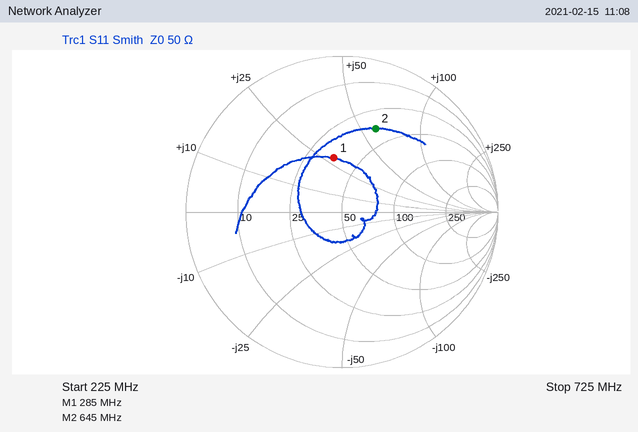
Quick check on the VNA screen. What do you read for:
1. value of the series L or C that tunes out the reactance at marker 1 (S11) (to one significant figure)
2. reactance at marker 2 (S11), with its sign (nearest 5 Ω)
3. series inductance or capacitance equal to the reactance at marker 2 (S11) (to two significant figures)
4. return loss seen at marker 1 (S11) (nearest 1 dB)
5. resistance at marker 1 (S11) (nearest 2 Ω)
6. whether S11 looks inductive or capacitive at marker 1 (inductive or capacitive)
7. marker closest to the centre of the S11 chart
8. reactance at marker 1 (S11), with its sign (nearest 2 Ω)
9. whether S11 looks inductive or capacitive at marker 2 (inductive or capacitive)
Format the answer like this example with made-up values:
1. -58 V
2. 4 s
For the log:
1. 20 pF
2. +60 Ω
3. 15 nH
4. 9 dB
5. 36 Ω
6. inductive
7. marker 1
8. +28 Ω
9. inductive
